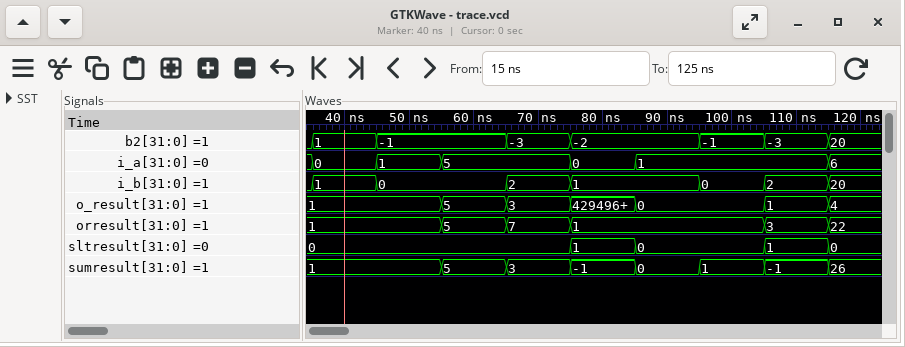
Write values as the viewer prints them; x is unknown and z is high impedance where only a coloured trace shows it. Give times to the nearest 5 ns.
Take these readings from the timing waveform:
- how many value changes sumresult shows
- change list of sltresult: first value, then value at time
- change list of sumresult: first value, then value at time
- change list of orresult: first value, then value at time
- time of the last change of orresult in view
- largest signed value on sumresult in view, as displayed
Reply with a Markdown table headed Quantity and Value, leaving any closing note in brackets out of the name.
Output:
| Quantity | Value |
|---|---|
| how many value changes sumresult shows | 7 |
| change list of sltresult: first value, then value at time | 0, 1 at 75 ns, 0 at 85 ns, 1 at 105 ns, 0 at 115 ns |
| change list of sumresult: first value, then value at time | 1, 5 at 55 ns, 3 at 65 ns, -1 at 75 ns, 0 at 85 ns, 1 at 95 ns, -1 at 105 ns, 26 at 115 ns |
| change list of orresult: first value, then value at time | 1, 5 at 55 ns, 7 at 65 ns, 1 at 75 ns, 3 at 105 ns, 22 at 115 ns |
| time of the last change of orresult in view | 115 ns |
| largest signed value on sumresult in view, as displayed | 26 |
